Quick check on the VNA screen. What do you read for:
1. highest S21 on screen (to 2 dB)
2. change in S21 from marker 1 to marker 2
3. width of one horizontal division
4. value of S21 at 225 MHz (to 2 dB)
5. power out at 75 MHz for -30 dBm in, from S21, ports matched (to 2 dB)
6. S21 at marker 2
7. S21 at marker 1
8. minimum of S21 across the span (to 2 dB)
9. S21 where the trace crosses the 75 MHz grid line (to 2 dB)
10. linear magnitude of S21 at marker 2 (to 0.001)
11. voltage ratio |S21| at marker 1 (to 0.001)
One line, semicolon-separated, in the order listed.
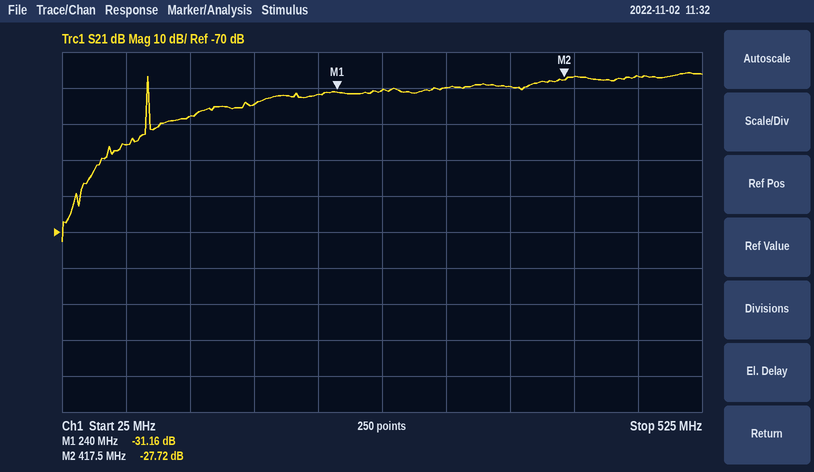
-26 dB; 3.44 dB; 50 MHz; -32 dB; -76 dBm; -27.72 dB; -31.16 dB; -72 dB; -46 dB; 0.041; 0.028
